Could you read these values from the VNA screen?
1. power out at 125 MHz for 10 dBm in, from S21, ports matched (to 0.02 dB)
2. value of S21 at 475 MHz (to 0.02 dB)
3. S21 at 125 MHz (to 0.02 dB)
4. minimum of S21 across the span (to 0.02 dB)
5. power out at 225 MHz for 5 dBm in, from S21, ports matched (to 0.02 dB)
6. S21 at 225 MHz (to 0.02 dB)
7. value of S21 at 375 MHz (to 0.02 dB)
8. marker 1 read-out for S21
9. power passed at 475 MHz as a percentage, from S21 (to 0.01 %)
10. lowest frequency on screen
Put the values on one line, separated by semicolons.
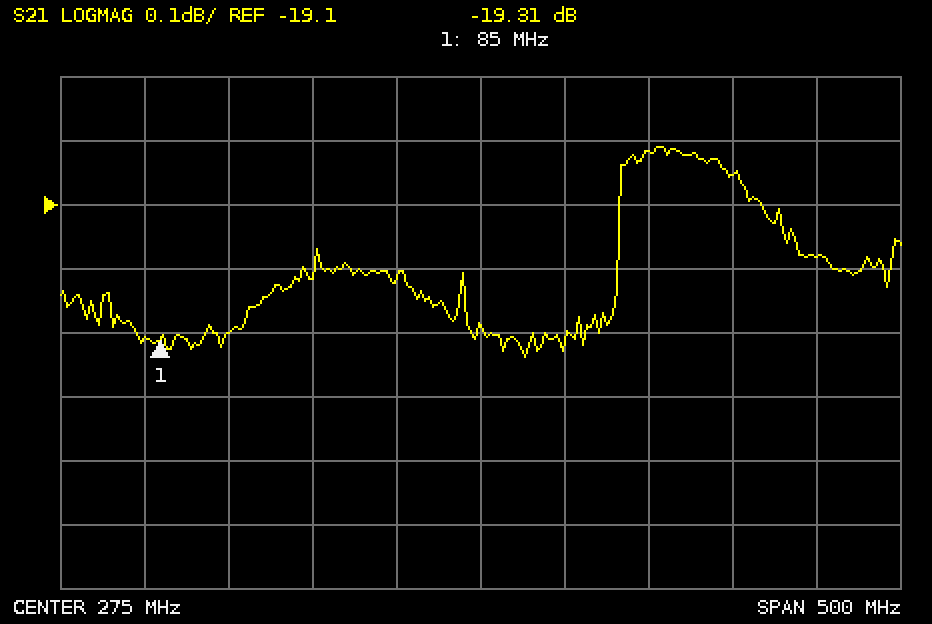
-9.30 dBm; -19.18 dB; -19.30 dB; -19.34 dB; -14.22 dBm; -19.22 dB; -19.02 dB; -19.31 dB; 1.21 %; 25 MHz
